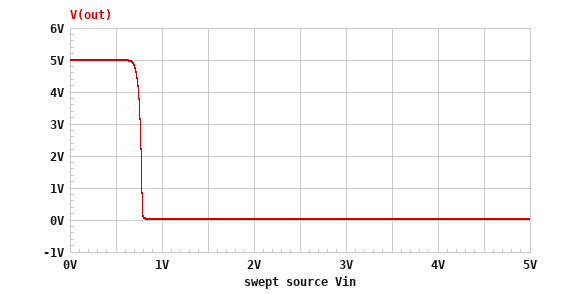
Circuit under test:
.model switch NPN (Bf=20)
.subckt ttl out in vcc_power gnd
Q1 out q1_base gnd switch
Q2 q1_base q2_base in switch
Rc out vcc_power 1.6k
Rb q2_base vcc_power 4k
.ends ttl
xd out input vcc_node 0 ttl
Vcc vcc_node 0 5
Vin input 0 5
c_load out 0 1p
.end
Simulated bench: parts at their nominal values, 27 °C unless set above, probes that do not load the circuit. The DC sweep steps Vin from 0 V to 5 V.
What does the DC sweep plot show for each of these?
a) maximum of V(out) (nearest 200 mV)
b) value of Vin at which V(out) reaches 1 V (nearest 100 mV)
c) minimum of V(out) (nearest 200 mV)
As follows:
5.0 V
800 mV
0 V
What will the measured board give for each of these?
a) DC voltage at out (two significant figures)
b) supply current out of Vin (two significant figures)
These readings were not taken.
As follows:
37 mV
850 µA
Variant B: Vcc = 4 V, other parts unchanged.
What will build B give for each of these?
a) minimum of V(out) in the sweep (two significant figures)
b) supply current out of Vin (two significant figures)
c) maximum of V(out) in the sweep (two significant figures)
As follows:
39 mV
610 µA
4.0 V
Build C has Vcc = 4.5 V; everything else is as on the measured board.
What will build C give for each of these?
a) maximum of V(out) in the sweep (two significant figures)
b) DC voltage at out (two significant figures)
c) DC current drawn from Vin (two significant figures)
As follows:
4.5 V
38 mV
730 µA
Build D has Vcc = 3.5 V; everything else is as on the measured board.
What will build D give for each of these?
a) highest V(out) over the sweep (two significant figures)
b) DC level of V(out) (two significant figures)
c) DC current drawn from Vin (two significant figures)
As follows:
3.5 V
40 mV
480 µA
